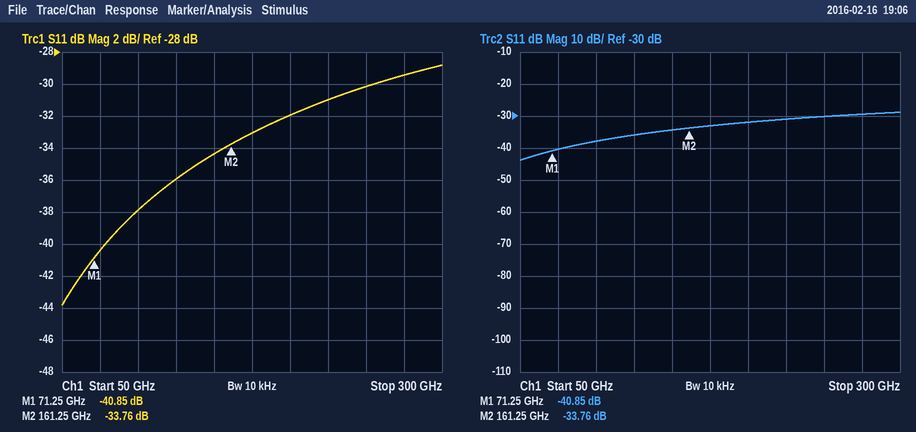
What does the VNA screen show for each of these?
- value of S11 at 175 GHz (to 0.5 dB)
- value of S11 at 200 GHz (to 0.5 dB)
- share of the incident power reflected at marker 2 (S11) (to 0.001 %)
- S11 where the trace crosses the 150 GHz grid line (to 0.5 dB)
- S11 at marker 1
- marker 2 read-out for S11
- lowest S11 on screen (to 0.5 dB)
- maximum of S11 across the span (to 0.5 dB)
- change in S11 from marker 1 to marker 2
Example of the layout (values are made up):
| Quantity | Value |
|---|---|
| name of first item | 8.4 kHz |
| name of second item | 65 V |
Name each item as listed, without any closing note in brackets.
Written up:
| Quantity | Value |
|---|---|
| value of S11 at 175 GHz | -33.0 dB |
| value of S11 at 200 GHz | -32.0 dB |
| share of the incident power reflected at marker 2 (S11) | 0.042 % |
| S11 where the trace crosses the 150 GHz grid line | -34.5 dB |
| S11 at marker 1 | -40.85 dB |
| marker 2 read-out for S11 | -33.76 dB |
| lowest S11 on screen | -44.0 dB |
| maximum of S11 across the span | -29.0 dB |
| change in S11 from marker 1 to marker 2 | 7.09 dB |
